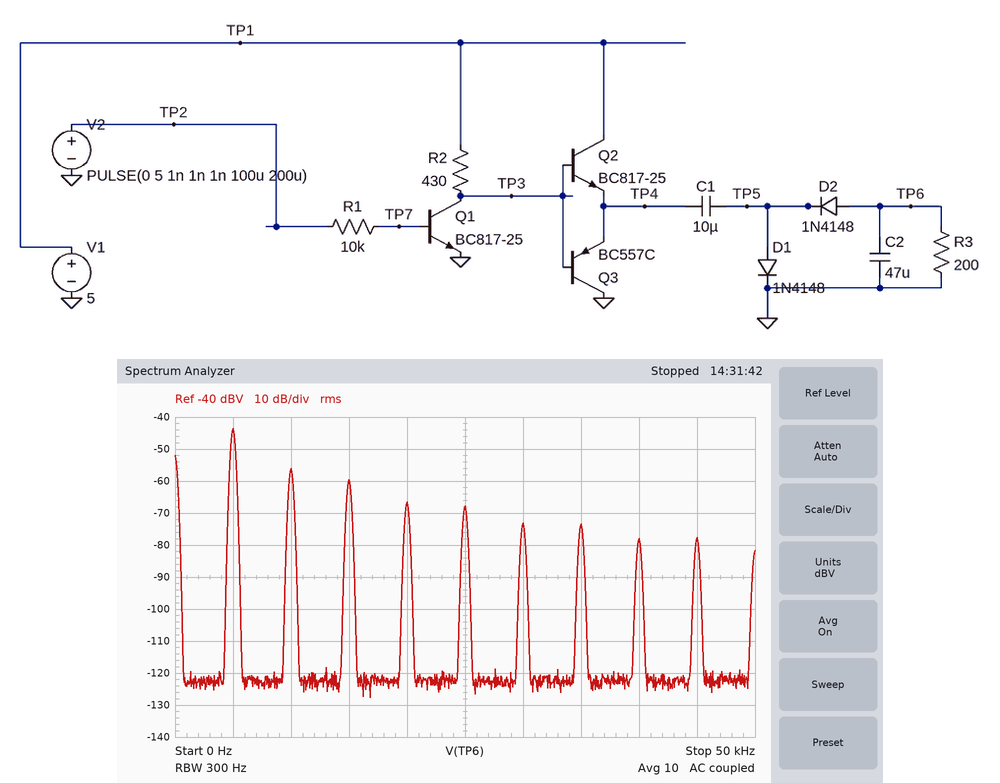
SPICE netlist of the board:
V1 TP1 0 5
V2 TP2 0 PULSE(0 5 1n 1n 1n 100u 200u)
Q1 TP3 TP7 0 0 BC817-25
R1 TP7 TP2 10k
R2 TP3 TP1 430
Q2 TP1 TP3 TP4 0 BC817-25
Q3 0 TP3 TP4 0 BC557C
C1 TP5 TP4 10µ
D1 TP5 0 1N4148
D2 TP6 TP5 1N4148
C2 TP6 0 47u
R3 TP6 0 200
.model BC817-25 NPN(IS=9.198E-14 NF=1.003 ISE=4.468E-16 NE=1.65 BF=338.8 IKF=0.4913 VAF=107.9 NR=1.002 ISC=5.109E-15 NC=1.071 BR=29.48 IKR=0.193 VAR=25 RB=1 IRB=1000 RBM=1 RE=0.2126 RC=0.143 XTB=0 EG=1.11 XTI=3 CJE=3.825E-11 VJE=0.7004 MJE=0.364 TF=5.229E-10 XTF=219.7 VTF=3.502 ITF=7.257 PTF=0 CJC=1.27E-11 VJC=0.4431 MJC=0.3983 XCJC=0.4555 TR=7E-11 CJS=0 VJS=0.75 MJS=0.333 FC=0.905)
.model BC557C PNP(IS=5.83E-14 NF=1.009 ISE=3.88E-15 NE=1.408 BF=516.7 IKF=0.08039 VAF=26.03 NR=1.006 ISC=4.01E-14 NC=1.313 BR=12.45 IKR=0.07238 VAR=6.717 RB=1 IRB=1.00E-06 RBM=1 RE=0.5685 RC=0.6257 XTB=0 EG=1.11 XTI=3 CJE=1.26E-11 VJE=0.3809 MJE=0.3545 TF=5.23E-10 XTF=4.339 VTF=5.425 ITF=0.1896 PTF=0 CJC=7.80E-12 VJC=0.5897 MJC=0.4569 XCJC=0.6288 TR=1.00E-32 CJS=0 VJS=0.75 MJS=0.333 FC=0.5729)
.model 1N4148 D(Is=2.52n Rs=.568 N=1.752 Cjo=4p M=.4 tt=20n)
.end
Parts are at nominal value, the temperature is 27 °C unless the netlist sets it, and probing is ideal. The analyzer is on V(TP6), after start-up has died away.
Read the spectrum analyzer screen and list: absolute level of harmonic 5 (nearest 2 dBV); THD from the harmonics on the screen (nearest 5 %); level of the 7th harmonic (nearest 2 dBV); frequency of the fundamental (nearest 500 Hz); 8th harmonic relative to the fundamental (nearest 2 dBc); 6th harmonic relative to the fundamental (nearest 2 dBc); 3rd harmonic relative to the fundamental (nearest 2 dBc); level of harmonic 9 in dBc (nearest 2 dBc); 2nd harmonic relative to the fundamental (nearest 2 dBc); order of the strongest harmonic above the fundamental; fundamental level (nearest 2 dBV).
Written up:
-68 dBV
30 %
-74 dBV
5.0 kHz
-34 dBc
-30 dBc
-16 dBc
-34 dBc
-12 dBc
2
-44 dBV
